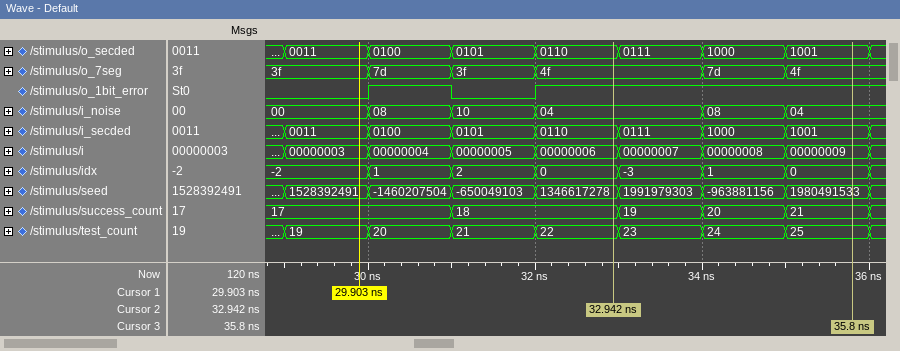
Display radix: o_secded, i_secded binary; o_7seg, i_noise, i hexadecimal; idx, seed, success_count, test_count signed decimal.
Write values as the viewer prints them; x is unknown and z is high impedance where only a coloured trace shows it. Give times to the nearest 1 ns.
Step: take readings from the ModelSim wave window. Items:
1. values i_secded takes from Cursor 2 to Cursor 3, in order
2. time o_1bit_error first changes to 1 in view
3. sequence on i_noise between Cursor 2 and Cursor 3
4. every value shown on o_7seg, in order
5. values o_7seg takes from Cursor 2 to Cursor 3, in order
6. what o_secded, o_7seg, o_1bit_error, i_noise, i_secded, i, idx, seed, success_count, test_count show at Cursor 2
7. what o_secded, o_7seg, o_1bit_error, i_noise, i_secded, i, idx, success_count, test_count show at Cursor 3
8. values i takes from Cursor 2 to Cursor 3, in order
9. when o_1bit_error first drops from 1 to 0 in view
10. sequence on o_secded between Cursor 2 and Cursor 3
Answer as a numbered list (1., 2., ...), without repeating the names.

1. 0110, 0111, 1000, 1001
2. 30 ns
3. 04, 08, 04
4. 3f, 7d, 3f, 4f, 7d, 4f
5. 4f, 7d, 4f
6. o_secded=0110, o_7seg=4f, o_1bit_error=1, i_noise=04, i_secded=0110, i=00000006, idx=0, seed=1346617278, success_count=18, test_count=22
7. o_secded=1001, o_7seg=4f, o_1bit_error=1, i_noise=04, i_secded=1001, i=00000009, idx=0, success_count=21, test_count=25
8. 00000006, 00000007, 00000008, 00000009
9. 31 ns
10. 0110, 0111, 1000, 1001
